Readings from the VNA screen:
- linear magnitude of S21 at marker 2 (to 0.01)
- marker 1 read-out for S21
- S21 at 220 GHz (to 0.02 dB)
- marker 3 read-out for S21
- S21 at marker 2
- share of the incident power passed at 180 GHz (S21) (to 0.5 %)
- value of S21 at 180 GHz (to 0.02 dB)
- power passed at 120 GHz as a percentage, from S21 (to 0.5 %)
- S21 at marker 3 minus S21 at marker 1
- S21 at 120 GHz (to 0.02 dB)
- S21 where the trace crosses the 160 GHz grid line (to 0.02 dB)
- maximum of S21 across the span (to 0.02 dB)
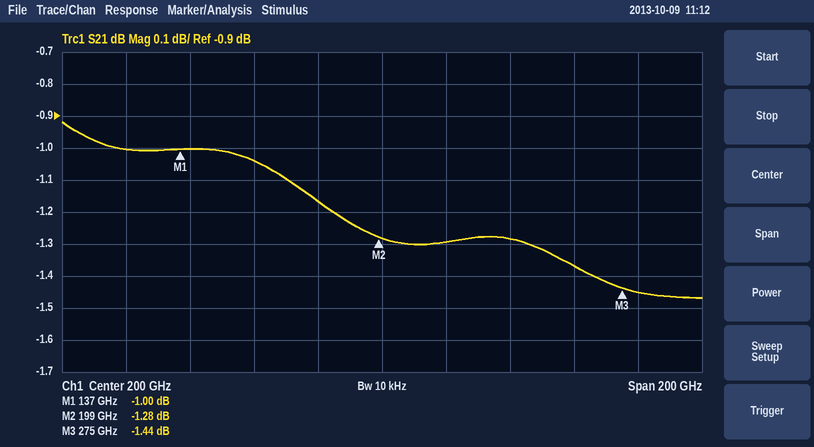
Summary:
0.86
-1.00 dB
-1.30 dB
-1.44 dB
-1.28 dB
76.5 %
-1.16 dB
79.5 %
-0.44 dB
-1.00 dB
-1.04 dB
-0.92 dB
